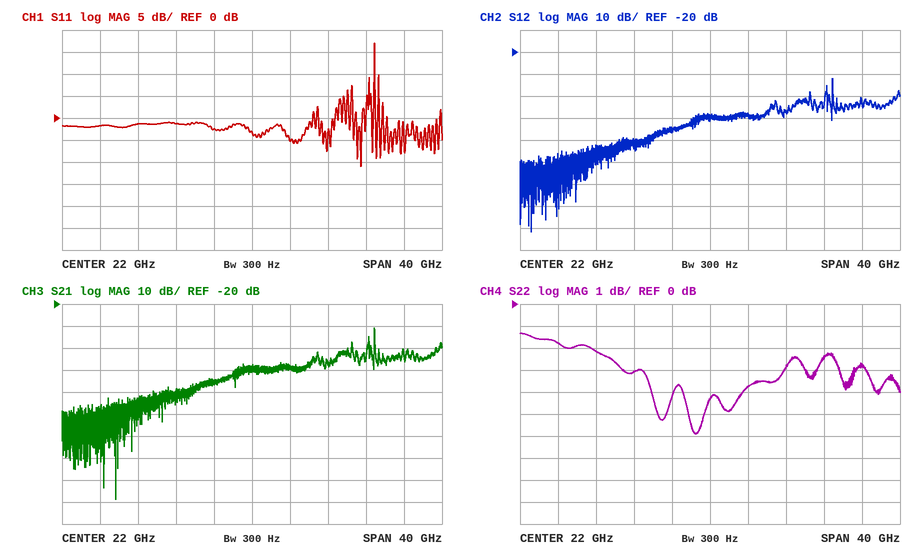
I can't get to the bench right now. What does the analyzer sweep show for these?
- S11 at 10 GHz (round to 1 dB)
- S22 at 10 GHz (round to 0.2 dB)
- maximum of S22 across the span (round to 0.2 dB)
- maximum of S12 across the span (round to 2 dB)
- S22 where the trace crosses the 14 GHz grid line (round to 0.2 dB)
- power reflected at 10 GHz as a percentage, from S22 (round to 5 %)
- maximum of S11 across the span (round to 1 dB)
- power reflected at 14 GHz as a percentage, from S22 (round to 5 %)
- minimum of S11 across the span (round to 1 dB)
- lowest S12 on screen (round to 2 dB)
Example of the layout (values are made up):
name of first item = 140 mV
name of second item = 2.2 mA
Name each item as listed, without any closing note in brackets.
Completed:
S11 at 10 GHz = -1 dB
S22 at 10 GHz = -2.2 dB
maximum of S22 across the span = -1.4 dB
maximum of S12 across the span = -32 dB
S22 where the trace crosses the 14 GHz grid line = -3.0 dB
power reflected at 10 GHz as a percentage, from S22 = 60 %
maximum of S11 across the span = 17 dB
power reflected at 14 GHz as a percentage, from S22 = 50 %
minimum of S11 across the span = -11 dB
lowest S12 on screen = -102 dB
